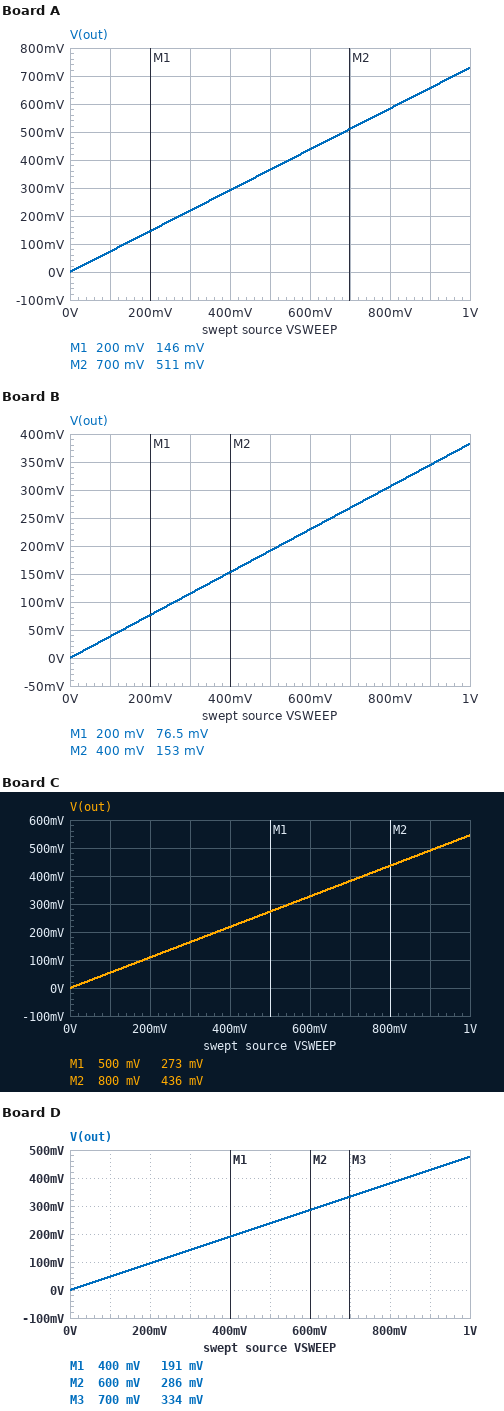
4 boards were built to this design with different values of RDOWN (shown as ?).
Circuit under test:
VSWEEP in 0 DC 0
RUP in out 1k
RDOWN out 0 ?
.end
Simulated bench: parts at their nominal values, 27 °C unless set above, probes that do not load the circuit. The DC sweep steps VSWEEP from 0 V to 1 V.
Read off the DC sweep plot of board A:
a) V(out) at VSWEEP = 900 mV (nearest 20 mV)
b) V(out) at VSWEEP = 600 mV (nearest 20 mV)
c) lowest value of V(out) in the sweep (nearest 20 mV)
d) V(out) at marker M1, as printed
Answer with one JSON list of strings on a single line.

["660 mV", "440 mV", "0 V", "146 mV"]
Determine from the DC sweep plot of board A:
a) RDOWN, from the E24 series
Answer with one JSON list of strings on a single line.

["2.7 kΩ"]
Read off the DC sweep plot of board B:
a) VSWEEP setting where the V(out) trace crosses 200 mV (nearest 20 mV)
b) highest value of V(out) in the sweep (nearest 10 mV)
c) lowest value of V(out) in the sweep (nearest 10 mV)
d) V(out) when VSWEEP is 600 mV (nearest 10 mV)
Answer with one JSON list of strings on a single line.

["520 mV", "380 mV", "0 V", "230 mV"]
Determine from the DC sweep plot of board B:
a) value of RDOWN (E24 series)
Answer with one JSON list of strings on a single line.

["620 Ω"]
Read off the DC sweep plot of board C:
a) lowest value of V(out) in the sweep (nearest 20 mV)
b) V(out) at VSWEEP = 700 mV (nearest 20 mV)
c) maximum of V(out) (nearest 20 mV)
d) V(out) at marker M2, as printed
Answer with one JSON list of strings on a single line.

["0 V", "380 mV", "540 mV", "436 mV"]
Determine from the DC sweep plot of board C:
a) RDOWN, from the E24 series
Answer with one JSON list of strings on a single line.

["1.2 kΩ"]
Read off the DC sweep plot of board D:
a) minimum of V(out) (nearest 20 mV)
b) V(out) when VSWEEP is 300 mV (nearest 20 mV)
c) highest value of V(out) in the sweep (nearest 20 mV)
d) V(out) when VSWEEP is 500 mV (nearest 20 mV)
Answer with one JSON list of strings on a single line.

["0 V", "140 mV", "480 mV", "240 mV"]
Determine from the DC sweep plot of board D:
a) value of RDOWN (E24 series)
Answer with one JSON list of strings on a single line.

["910 Ω"]
